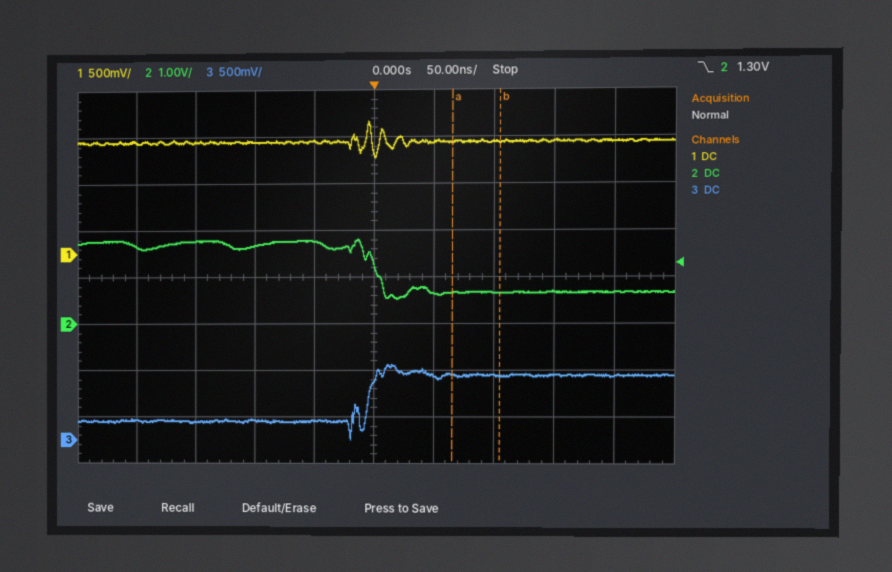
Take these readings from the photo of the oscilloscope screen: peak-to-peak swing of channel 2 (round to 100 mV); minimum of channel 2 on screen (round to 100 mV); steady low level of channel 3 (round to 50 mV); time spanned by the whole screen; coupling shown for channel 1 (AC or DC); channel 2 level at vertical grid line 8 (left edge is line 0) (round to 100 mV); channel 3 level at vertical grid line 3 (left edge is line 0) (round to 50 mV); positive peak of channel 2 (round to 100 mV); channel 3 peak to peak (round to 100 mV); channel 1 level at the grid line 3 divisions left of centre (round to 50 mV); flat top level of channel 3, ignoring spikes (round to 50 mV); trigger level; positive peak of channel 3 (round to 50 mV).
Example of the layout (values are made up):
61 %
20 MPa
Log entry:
1.3 V
500 mV
200 mV
500 ns
DC
700 mV
200 mV
1.8 V
800 mV
1.20 V
700 mV
1.30 V
800 mV
